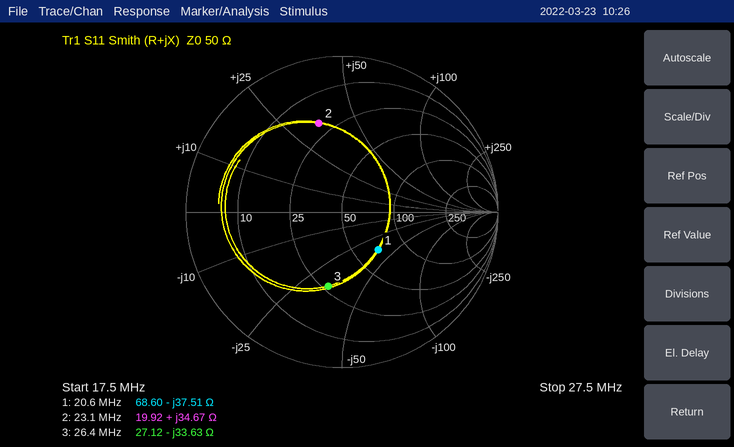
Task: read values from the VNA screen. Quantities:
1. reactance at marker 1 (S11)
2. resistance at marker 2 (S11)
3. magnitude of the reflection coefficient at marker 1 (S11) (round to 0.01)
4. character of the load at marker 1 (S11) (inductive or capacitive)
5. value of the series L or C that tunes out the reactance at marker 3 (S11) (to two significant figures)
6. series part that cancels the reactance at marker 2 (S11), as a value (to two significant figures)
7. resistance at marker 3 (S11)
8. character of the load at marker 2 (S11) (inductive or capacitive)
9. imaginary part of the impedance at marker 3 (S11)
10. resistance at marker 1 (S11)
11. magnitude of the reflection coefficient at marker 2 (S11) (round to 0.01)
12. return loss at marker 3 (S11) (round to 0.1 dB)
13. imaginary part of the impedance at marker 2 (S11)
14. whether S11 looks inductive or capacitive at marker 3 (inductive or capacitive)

-37.51 Ω
19.92 Ω
0.34
capacitive
200 nH
200 pF
27.12 Ω
inductive
-33.63 Ω
68.60 Ω
0.59
6.3 dB
+34.67 Ω
capacitive
